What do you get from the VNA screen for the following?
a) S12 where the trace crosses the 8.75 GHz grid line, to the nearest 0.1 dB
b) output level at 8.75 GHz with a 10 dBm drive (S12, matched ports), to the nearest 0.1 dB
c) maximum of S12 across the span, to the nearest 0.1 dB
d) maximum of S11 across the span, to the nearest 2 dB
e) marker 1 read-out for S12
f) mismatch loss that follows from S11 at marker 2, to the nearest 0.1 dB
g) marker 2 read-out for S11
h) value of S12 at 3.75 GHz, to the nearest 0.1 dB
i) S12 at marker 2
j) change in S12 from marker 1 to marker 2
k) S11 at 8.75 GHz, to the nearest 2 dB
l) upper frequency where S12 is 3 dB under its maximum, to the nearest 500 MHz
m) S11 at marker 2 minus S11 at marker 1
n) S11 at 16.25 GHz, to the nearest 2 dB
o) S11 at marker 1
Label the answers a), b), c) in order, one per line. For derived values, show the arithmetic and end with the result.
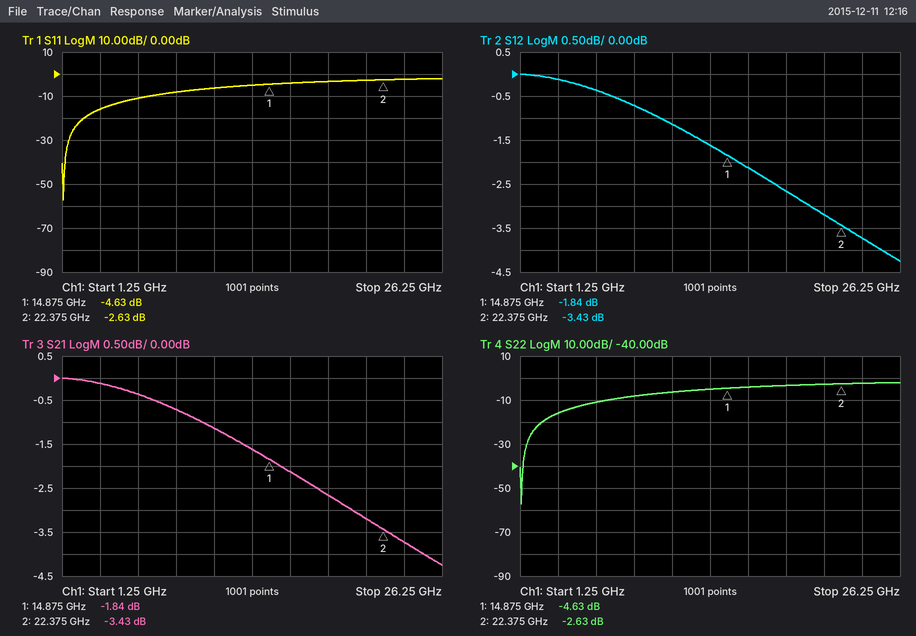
a) -0.7 dB
b) 10 dBm + (-0.7 dB) = 9.3 dBm
c) 0.0 dB
d) -2 dB
e) -1.84 dB
f) −10 log10(1 − 10^(-2.63/10)) ≈ 3.4 dB
g) -2.63 dB
h) -0.1 dB
i) -3.43 dB
j) -3.43 − (-1.84) = -1.59 dB
k) -8 dB
l) 20.5 GHz
m) -2.63 − (-4.63) = 2.00 dB
n) -4 dB
o) -4.63 dB
